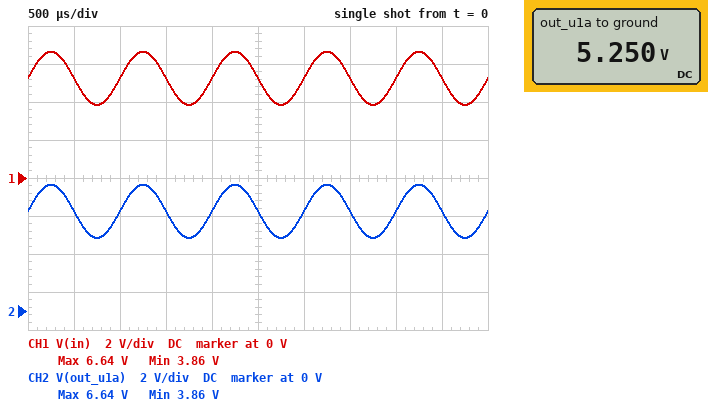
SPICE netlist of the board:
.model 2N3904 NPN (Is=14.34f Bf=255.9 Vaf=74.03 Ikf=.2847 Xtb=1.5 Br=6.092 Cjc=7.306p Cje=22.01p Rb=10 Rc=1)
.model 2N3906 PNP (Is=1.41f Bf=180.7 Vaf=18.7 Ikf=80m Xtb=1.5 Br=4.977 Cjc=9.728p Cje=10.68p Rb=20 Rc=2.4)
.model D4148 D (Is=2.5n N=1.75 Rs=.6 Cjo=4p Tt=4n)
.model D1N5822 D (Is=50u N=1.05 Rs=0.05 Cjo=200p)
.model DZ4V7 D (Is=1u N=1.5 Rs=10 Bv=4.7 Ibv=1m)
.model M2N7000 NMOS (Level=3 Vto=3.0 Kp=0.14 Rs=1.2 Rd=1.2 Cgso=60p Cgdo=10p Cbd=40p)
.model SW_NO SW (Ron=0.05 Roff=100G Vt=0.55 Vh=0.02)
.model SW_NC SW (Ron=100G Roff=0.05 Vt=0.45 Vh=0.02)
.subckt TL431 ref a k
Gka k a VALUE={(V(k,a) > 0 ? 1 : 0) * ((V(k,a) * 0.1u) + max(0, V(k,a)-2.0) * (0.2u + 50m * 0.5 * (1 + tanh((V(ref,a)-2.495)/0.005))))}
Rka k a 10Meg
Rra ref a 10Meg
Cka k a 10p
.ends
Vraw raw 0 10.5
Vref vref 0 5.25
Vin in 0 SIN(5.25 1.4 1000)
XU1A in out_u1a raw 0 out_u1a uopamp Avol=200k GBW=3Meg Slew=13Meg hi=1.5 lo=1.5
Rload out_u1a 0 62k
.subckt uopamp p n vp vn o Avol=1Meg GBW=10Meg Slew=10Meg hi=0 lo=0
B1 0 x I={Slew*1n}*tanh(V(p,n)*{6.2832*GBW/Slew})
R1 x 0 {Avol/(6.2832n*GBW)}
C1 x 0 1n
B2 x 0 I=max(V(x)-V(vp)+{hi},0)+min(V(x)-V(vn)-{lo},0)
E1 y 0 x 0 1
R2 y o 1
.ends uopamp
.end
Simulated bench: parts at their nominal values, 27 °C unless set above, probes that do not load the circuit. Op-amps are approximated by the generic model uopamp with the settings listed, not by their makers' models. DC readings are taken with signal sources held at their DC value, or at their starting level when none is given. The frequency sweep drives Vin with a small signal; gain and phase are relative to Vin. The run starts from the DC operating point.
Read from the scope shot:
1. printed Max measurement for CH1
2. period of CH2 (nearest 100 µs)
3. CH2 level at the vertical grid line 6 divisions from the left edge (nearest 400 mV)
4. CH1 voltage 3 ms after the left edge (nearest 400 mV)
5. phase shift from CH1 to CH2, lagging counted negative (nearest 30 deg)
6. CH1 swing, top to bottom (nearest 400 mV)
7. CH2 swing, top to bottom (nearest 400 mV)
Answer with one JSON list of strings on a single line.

["6.64 V", "1.0 ms", "5.2 V", "5.2 V", "0 deg", "2.8 V", "2.8 V"]
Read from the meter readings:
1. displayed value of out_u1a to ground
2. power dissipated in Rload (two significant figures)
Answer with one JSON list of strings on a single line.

["5.250 V", "440 µW"]
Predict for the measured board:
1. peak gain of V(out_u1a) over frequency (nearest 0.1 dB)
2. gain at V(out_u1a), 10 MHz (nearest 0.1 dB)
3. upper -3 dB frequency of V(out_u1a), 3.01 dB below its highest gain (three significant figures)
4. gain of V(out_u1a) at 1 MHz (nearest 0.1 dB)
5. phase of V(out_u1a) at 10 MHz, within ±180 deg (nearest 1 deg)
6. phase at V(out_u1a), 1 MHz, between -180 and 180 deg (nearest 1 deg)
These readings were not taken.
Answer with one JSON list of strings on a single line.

["0 dB", "-10.8 dB", "3.00 MHz", "-0.5 dB", "-73 deg", "-18 deg"]
